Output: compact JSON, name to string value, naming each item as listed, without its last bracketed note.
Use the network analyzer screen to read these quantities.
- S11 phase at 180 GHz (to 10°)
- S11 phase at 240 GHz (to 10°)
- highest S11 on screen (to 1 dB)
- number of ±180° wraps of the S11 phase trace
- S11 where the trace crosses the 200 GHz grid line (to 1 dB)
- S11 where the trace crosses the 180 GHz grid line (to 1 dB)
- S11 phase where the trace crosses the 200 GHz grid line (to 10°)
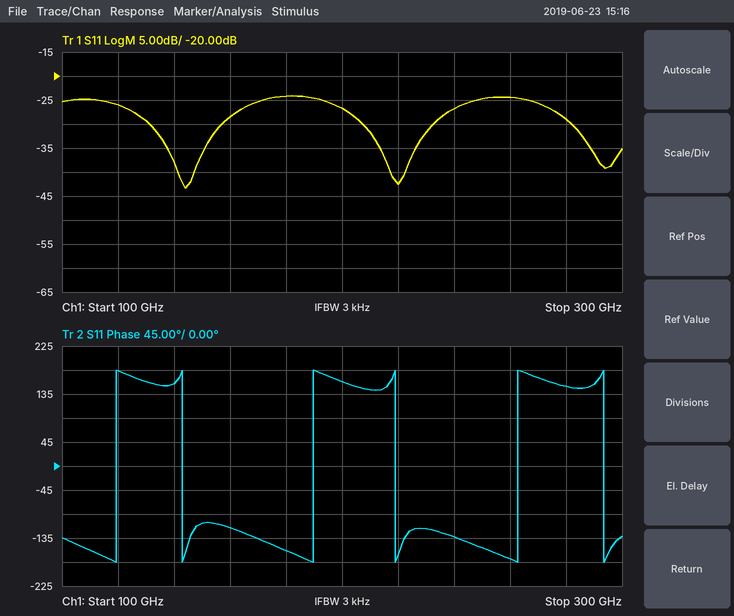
{"S11 phase at 180 GHz": "-160°", "S11 phase at 240 GHz": "-130°", "highest S11 on screen": "-24 dB", "number of ±180° wraps of the S11 phase trace": "6", "S11 where the trace crosses the 200 GHz grid line": "-27 dB", "S11 where the trace crosses the 180 GHz grid line": "-24 dB", "S11 phase where the trace crosses the 200 GHz grid line": "160°"}
